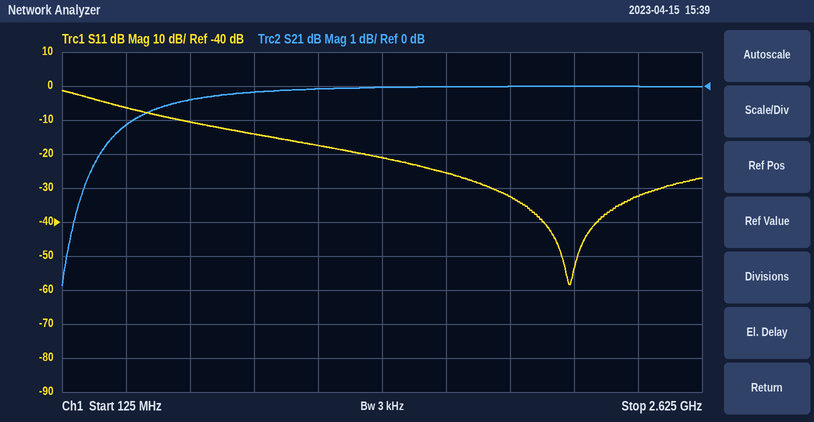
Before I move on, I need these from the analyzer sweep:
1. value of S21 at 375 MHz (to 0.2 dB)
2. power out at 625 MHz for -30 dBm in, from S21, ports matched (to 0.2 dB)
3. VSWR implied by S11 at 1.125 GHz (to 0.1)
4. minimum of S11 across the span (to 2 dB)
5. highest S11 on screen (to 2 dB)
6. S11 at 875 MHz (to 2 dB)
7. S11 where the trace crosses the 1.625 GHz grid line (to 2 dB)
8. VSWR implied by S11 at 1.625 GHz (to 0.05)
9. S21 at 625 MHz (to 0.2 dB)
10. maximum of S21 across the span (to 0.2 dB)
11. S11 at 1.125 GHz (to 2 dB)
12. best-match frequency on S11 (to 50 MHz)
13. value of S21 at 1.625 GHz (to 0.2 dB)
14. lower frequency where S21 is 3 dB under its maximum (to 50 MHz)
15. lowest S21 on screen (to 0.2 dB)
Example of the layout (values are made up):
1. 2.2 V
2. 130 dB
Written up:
1. -1.2 dB
2. -30.4 dBm
3. 1.3
4. -58 dB
5. -2 dB
6. -14 dB
7. -26 dB
8. 1.10
9. -0.4 dB
10. 0.0 dB
11. -18 dB
12. 2.10 GHz
13. 0.0 dB
14. 200 MHz
15. -5.8 dB
